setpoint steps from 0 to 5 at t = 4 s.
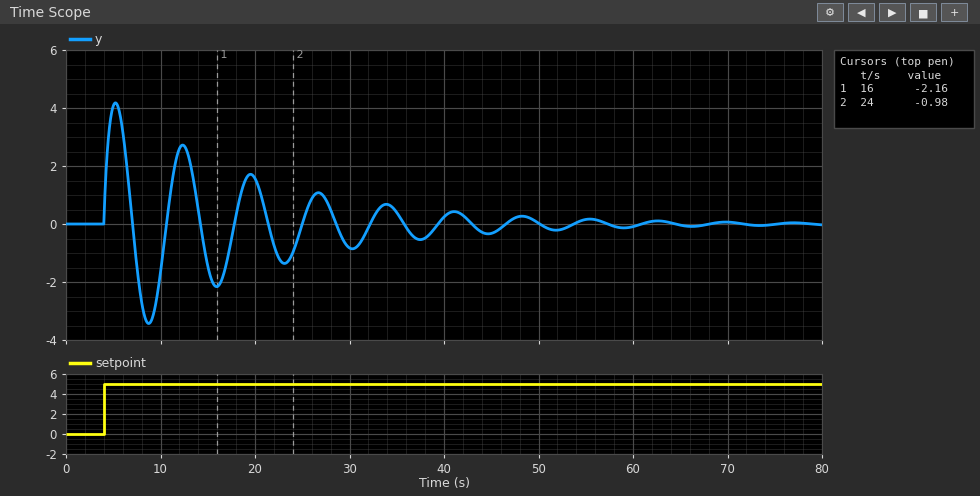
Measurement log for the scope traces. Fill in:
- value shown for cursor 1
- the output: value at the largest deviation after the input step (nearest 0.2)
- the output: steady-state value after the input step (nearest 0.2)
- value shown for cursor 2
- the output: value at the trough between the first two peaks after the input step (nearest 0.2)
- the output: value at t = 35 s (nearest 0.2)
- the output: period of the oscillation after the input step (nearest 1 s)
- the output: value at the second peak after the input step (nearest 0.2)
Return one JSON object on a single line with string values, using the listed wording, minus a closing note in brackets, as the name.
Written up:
{"value shown for cursor 1": "-2.16", "the output: value at the largest deviation after the input step": "4.2", "the output: steady-state value after the input step": "0.0", "value shown for cursor 2": "-0.98", "the output: value at the trough between the first two peaks after the input step": "-3.4", "the output: value at t = 35 s": "0.4", "the output: period of the oscillation after the input step": "7 s", "the output: value at the second peak after the input step": "2.8"}
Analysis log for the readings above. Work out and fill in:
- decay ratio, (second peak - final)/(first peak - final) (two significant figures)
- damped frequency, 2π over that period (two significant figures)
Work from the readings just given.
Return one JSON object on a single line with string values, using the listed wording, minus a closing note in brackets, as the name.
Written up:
{"decay ratio, (second peak - final)/(first peak - final)": "0.67", "damped frequency, 2π over that period": "0.90 rad/s"}
